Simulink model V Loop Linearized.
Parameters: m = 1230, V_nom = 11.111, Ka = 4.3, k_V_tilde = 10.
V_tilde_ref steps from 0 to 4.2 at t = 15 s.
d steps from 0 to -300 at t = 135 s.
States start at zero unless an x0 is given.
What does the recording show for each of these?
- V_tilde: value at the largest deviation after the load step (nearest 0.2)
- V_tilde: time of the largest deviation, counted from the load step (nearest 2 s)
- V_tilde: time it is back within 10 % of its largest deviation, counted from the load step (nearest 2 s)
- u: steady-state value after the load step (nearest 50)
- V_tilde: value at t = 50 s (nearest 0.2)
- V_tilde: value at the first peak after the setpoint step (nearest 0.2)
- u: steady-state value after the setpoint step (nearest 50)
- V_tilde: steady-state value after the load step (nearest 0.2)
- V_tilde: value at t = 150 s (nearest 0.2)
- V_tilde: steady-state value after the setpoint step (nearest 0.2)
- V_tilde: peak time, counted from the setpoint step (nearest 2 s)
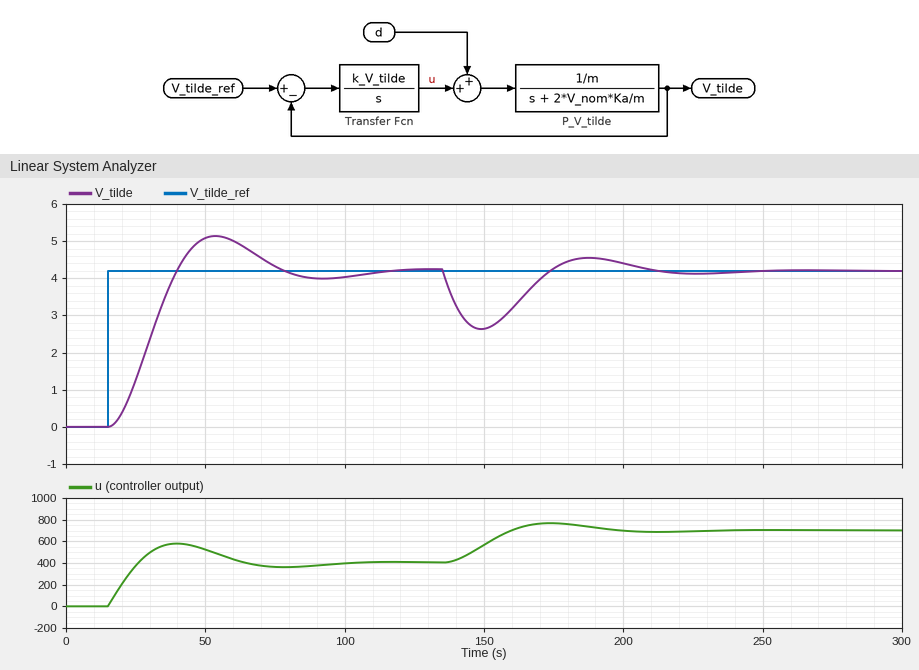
2.6
14 s
68 s
700
5.0
5.2
400
4.2
2.6
4.2
38 s
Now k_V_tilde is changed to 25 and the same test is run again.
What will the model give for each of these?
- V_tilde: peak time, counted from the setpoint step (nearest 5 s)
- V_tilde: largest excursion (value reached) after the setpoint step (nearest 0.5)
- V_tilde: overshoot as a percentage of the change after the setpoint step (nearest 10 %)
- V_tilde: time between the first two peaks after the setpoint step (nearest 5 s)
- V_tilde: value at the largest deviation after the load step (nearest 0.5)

25 s
6.0
40 %
45 s
3.0
